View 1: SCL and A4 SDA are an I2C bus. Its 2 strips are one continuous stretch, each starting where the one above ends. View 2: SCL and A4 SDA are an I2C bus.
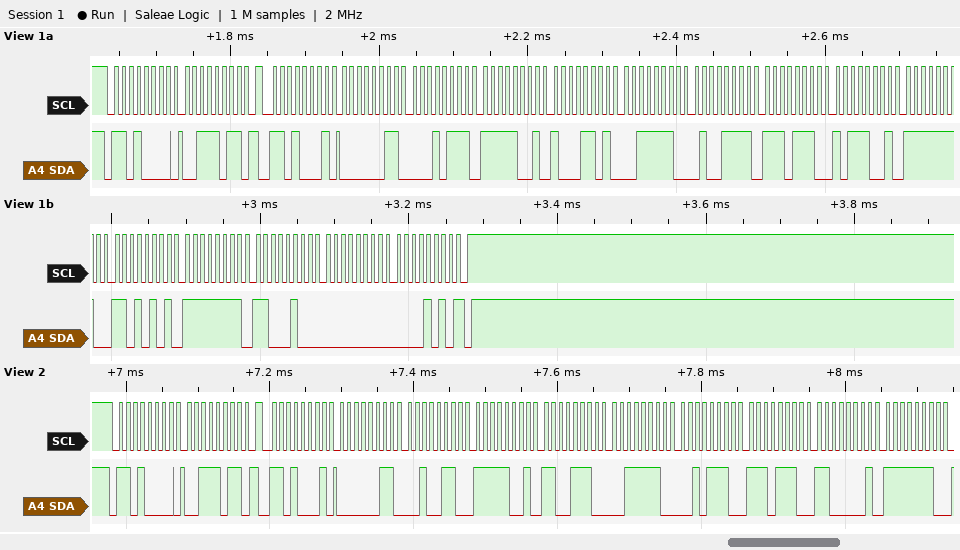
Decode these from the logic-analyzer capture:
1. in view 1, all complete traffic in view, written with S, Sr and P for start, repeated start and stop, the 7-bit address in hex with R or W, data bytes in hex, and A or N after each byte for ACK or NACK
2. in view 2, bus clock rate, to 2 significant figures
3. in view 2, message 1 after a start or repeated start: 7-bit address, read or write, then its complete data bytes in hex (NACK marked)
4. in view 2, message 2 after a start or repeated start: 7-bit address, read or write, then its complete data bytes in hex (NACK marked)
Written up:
S 68W A 3B A Sr 68R A 03 A 17 A F9 A 8D A 3E A 4F A EE A B9 A FE A D5 A FF A C4 A 00 A 0A N P
100 kHz
0x68 write: 3B
0x68 read: 03 26 F9 CE 3E 2E EE C1 FE
